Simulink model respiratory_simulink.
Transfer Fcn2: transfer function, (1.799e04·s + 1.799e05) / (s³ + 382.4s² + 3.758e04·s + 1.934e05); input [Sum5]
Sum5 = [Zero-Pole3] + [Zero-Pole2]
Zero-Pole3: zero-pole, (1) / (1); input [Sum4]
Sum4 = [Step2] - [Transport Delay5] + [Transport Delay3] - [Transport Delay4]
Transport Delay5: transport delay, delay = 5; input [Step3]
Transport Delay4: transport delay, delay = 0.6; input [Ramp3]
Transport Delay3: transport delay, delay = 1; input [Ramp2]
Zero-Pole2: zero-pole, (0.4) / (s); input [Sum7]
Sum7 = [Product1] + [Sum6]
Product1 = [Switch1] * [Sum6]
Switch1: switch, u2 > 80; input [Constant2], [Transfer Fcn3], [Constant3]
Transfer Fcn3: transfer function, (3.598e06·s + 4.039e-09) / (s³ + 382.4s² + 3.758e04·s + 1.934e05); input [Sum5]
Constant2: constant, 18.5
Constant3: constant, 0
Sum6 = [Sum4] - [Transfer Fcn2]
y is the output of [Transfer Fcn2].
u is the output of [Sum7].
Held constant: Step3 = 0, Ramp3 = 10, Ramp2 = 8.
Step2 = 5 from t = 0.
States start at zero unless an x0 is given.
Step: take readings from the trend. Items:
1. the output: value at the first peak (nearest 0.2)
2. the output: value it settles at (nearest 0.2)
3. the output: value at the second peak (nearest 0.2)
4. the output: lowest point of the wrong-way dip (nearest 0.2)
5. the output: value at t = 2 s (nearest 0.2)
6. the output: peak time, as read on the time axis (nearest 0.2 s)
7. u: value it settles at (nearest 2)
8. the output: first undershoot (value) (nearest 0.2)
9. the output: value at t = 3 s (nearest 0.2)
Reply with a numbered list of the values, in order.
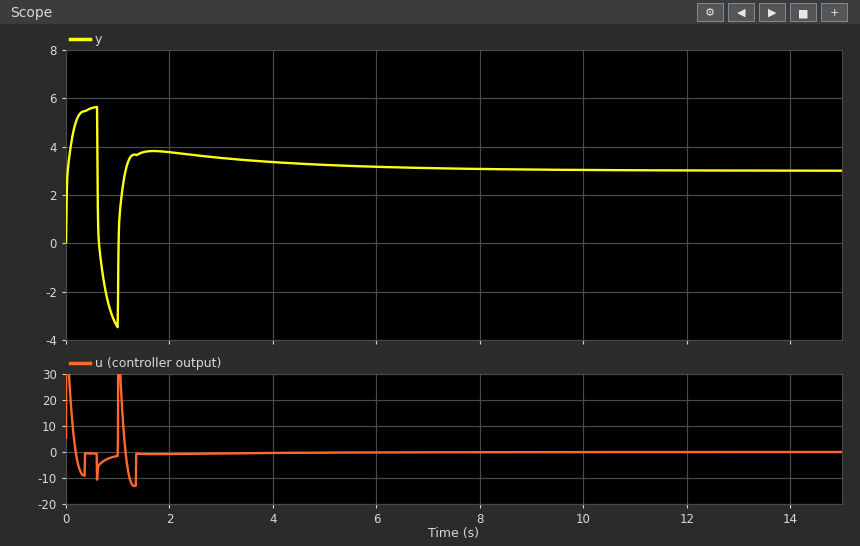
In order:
1. 5.6
2. 3.0
3. 3.8
4. -3.4
5. 3.8
6. 0.6 s
7. 0
8. -3.4
9. 3.6
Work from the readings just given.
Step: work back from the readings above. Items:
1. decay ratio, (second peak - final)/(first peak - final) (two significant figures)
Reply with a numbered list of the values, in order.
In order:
1. 0.31
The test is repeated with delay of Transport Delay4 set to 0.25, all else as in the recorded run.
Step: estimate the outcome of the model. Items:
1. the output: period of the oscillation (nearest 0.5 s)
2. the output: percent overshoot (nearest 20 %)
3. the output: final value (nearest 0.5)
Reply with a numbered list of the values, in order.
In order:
1. 1.5 s
2. 80 %
3. 3.0
